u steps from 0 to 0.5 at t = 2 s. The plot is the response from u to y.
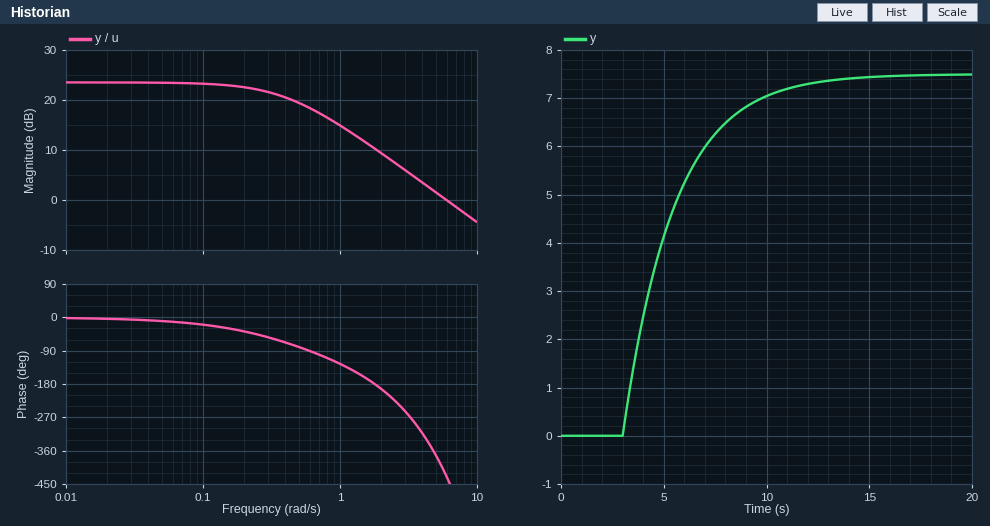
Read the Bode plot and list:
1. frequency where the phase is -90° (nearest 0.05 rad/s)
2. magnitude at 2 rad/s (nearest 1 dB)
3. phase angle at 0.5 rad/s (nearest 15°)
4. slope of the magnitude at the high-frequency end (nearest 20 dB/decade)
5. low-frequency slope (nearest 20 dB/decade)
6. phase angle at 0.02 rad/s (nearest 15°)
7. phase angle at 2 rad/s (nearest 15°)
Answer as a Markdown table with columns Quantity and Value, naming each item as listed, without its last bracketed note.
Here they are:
| Quantity | Value |
|---|---|
| frequency where the phase is -90° | 0.60 rad/s |
| magnitude at 2 rad/s | 9 dB |
| phase angle at 0.5 rad/s | -75° |
| slope of the magnitude at the high-frequency end | -20 dB/decade |
| low-frequency slope | 0 dB/decade |
| phase angle at 0.02 rad/s | 0° |
| phase angle at 2 rad/s | -195° |
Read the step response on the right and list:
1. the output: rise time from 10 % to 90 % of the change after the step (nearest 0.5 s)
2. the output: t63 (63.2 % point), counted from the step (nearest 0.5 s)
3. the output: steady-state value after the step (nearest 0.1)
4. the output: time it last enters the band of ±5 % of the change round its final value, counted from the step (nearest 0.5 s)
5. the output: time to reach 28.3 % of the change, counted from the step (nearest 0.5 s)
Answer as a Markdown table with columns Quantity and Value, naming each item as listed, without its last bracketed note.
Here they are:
| Quantity | Value |
|---|---|
| the output: rise time from 10 % to 90 % of the change after the step | 5.5 s |
| the output: t63 (63.2 % point), counted from the step | 3.5 s |
| the output: steady-state value after the step | 7.5 |
| the output: time it last enters the band of ±5 % of the change round its final value, counted from the step | 8.5 s |
| the output: time to reach 28.3 % of the change, counted from the step | 2.0 s |
